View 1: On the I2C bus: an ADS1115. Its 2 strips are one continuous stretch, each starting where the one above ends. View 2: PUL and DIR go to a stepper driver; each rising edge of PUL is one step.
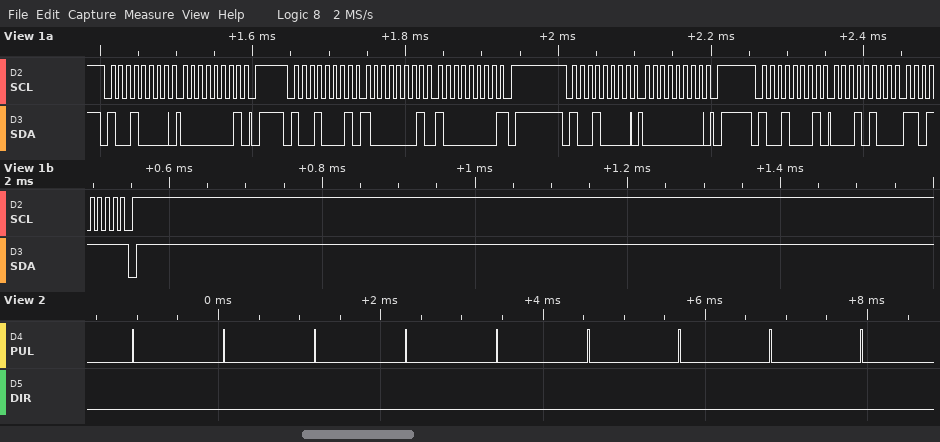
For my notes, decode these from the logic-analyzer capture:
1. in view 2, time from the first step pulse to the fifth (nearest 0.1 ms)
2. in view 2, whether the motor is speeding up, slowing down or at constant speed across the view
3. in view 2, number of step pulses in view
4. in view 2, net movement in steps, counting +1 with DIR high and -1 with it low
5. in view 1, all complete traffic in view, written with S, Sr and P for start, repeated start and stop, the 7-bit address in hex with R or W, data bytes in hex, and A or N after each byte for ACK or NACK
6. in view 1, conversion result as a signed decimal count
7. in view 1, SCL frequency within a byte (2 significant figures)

4.5 ms
constant speed
9
-9
S 48W A 01 A P S 48R A 81 A 80 N P S 48W A 00 A P S 48R A 14 A DF N P
5343
100 kHz
